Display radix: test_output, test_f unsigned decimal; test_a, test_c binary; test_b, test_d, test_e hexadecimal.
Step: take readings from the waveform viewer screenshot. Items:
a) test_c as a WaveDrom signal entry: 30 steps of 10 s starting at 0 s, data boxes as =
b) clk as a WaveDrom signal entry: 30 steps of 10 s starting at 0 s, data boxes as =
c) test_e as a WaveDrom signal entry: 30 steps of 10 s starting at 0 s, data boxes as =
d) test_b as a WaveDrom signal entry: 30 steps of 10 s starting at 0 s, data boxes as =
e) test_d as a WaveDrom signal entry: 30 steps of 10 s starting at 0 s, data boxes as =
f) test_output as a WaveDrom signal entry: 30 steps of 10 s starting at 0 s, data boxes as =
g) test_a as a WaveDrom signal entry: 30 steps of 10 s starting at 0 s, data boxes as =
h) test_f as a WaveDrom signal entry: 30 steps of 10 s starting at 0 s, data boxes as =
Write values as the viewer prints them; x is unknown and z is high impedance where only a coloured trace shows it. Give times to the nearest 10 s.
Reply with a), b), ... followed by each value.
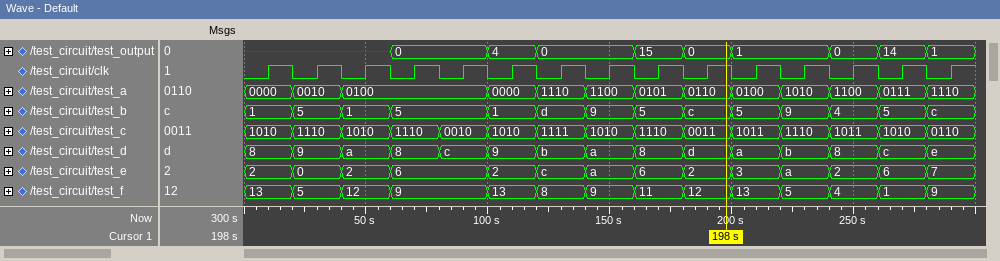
a) {name: 'test_c', wave: '=.=.=.=.=.=.=.=.=.=.=.=.=.=.=.', data: '1010 1110 1010 1110 0010 1010 1111 1010 1110 0011 1011 1110 1011 1010 0110'}
b) {name: 'clk', wave: '010101010101010101010101010101'}
c) {name: 'test_e', wave: '=.=.=.=...=.=.=.=.=.=.=.=.=.=.', data: '2 0 2 6 2 c a 6 2 3 a 2 6 7'}
d) {name: 'test_b', wave: '=.=.=.=...=.=.=.=.=.=.=.=.=.=.', data: '1 5 1 5 1 d 9 5 c 5 9 4 5 c'}
e) {name: 'test_d', wave: '=.=.=.=.=.=.=.=.=.=.=.=.=.=.=.', data: '8 9 a 8 c 9 b a 8 d a b 8 c e'}
f) {name: 'test_output', wave: 'x.....=...=.=...=.=.=...=.=.=.', data: '0 4 0 15 0 1 0 14 1'}
g) {name: 'test_a', wave: '=.=.=.....=.=.=.=.=.=.=.=.=.=.', data: '0000 0010 0100 0000 1110 1100 0101 0110 0100 1010 1100 0111 1110'}
h) {name: 'test_f', wave: '=.=.=.=...=.=.=.=.=.=.=.=.=.=.', data: '13 5 12 9 13 8 9 11 12 13 5 4 1 9'}
